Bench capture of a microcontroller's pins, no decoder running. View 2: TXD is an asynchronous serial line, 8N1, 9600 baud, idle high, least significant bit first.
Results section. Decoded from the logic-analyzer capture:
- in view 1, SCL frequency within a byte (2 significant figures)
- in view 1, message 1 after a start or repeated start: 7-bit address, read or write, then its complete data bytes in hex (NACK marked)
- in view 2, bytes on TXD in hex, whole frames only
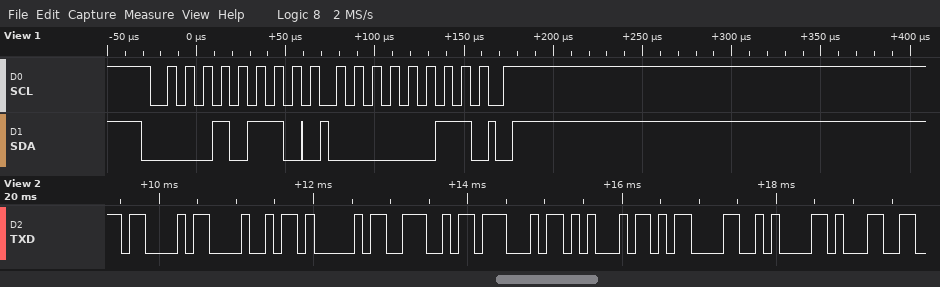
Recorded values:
100 kHz
0x0B write: 03
43 48 41 4E 47 45 0D 0A 31
